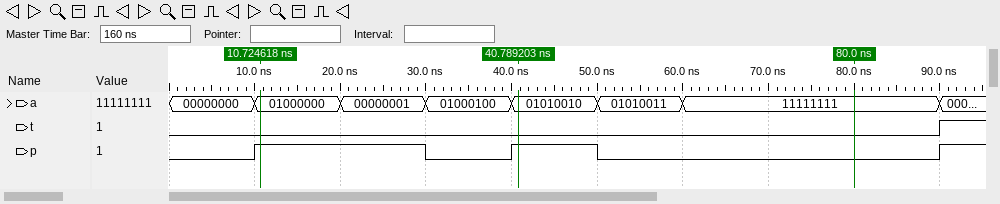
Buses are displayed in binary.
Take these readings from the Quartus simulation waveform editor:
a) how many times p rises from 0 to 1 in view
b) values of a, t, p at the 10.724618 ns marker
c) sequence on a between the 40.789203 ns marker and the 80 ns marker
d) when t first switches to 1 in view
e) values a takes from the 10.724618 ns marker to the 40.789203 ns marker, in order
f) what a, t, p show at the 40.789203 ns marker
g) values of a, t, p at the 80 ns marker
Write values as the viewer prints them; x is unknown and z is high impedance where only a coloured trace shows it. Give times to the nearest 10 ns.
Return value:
3
a=01000000, t=0, p=1
01010010, 01010011, 11111111
90 ns
01000000, 00000001, 01000100, 01010010
a=01010010, t=0, p=1
a=11111111, t=0, p=0
